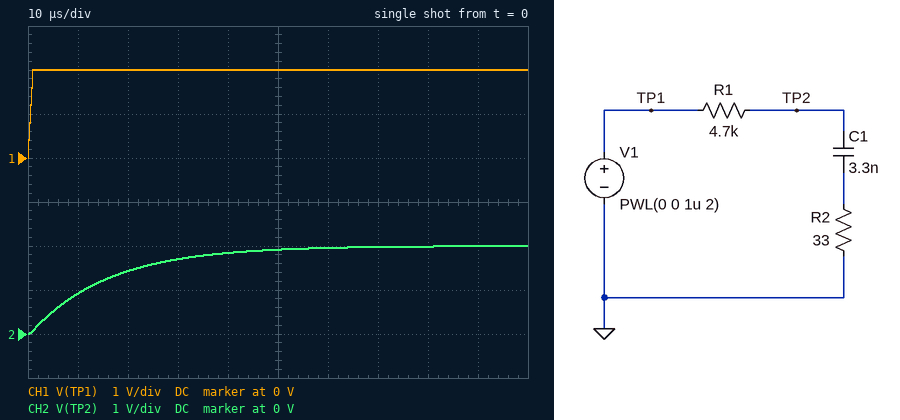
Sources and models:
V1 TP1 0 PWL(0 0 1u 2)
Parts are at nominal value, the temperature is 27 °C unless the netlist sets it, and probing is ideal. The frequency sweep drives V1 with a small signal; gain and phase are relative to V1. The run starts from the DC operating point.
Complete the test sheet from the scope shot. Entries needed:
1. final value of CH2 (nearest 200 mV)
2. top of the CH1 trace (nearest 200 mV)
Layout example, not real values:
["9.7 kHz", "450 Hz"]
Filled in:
["2.0 V", "2.0 V"]
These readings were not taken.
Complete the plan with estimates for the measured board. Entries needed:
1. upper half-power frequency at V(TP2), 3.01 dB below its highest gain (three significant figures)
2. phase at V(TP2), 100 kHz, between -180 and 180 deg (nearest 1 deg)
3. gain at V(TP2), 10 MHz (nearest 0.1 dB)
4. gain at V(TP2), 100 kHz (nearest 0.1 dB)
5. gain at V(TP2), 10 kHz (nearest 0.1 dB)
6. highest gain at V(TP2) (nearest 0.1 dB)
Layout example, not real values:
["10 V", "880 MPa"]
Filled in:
["10.2 kHz", "-80 deg", "-43.0 dB", "-19.9 dB", "-2.9 dB", "0 dB"]
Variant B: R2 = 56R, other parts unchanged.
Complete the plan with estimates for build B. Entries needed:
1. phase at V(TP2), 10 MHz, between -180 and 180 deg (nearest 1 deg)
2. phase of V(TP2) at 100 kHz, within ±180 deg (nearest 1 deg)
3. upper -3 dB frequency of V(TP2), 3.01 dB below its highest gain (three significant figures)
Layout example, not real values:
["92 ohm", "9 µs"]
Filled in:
["-5 deg", "-78 deg", "10.1 kHz"]
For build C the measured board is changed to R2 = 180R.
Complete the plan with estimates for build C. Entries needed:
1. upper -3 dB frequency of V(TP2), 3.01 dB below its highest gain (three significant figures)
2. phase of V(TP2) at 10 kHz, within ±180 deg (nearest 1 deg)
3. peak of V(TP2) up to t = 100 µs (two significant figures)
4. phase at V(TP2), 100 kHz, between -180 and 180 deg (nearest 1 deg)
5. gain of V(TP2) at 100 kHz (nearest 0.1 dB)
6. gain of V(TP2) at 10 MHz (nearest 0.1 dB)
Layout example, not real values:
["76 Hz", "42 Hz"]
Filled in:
["9.90 kHz", "-43 deg", "2.0 V", "-64 deg", "-19.6 dB", "-28.7 dB"]
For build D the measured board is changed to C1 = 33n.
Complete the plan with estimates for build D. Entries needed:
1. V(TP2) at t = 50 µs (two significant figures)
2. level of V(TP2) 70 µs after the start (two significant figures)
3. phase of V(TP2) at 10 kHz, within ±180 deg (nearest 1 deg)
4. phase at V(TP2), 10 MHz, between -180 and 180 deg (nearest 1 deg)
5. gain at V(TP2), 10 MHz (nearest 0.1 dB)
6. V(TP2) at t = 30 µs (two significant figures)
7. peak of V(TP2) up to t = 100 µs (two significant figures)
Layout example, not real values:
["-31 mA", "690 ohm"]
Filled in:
["550 mV", "730 mV", "-80 deg", "-1 deg", "-43.1 dB", "360 mV", "950 mV"]
